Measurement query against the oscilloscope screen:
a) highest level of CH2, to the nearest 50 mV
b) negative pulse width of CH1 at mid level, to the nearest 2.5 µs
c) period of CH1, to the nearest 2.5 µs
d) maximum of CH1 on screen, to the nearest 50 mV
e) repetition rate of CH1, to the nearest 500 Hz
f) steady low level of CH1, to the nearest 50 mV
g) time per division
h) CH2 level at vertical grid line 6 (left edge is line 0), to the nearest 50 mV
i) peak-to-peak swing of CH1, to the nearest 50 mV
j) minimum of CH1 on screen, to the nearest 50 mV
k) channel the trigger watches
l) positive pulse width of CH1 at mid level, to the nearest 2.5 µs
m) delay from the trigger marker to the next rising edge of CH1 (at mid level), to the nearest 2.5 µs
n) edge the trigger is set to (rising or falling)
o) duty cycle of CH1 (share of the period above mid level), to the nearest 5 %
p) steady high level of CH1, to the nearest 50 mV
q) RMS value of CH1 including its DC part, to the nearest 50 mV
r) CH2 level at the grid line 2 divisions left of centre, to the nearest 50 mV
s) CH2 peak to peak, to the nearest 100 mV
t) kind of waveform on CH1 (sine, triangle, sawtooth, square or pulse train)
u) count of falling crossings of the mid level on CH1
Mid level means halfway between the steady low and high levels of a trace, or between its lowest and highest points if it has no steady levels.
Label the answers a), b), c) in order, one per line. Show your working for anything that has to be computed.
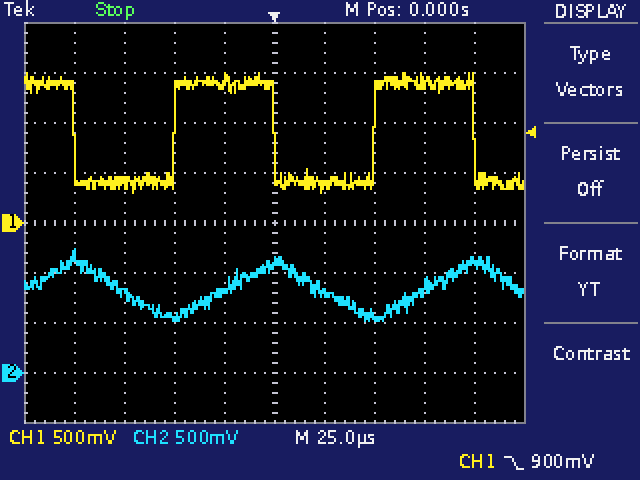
a) 1.25 V
b) 50.0 µs
c) 100.0 µs
d) 1.50 V
e) 1 / 100.0 µs ≈ 10.0 kHz
f) 400 mV
g) 25 µs
h) 800 mV
i) 1.50 V − (300 mV) = 1.20 V
j) 300 mV
k) CH1
l) 50.0 µs
m) 50.0 µs
n) falling
o) 50.0 µs / 100.0 µs ≈ 50 %
p) 1.40 V
q) √(0.5 × (1.40 V)² + 0.5 × (400 mV)²) ≈ 1.03 V, so 1.05 V to the nearest 50 mV
r) 550 mV
s) 700 mV
t) square
u) 3
